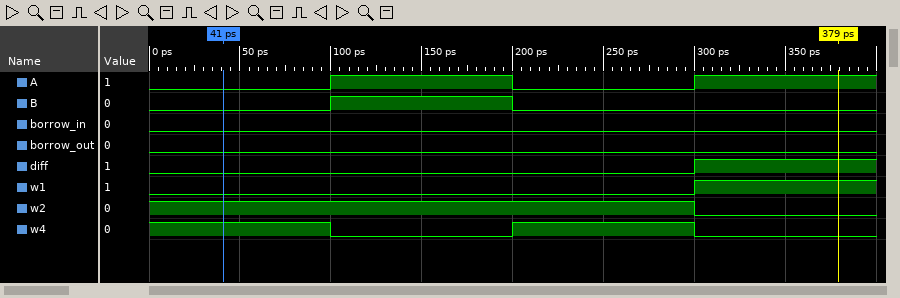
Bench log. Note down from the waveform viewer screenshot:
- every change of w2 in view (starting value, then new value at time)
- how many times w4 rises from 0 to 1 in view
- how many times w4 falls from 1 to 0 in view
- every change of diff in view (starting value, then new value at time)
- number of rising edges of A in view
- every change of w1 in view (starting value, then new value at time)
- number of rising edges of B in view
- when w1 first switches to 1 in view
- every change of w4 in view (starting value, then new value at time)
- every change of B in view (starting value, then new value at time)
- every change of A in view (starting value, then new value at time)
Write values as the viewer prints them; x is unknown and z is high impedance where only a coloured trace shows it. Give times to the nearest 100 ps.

1, 0 at 300 ps
1
2
0, 1 at 300 ps
2
0, 1 at 300 ps
1
300 ps
1, 0 at 100 ps, 1 at 200 ps, 0 at 300 ps
0, 1 at 100 ps, 0 at 200 ps
0, 1 at 100 ps, 0 at 200 ps, 1 at 300 ps
